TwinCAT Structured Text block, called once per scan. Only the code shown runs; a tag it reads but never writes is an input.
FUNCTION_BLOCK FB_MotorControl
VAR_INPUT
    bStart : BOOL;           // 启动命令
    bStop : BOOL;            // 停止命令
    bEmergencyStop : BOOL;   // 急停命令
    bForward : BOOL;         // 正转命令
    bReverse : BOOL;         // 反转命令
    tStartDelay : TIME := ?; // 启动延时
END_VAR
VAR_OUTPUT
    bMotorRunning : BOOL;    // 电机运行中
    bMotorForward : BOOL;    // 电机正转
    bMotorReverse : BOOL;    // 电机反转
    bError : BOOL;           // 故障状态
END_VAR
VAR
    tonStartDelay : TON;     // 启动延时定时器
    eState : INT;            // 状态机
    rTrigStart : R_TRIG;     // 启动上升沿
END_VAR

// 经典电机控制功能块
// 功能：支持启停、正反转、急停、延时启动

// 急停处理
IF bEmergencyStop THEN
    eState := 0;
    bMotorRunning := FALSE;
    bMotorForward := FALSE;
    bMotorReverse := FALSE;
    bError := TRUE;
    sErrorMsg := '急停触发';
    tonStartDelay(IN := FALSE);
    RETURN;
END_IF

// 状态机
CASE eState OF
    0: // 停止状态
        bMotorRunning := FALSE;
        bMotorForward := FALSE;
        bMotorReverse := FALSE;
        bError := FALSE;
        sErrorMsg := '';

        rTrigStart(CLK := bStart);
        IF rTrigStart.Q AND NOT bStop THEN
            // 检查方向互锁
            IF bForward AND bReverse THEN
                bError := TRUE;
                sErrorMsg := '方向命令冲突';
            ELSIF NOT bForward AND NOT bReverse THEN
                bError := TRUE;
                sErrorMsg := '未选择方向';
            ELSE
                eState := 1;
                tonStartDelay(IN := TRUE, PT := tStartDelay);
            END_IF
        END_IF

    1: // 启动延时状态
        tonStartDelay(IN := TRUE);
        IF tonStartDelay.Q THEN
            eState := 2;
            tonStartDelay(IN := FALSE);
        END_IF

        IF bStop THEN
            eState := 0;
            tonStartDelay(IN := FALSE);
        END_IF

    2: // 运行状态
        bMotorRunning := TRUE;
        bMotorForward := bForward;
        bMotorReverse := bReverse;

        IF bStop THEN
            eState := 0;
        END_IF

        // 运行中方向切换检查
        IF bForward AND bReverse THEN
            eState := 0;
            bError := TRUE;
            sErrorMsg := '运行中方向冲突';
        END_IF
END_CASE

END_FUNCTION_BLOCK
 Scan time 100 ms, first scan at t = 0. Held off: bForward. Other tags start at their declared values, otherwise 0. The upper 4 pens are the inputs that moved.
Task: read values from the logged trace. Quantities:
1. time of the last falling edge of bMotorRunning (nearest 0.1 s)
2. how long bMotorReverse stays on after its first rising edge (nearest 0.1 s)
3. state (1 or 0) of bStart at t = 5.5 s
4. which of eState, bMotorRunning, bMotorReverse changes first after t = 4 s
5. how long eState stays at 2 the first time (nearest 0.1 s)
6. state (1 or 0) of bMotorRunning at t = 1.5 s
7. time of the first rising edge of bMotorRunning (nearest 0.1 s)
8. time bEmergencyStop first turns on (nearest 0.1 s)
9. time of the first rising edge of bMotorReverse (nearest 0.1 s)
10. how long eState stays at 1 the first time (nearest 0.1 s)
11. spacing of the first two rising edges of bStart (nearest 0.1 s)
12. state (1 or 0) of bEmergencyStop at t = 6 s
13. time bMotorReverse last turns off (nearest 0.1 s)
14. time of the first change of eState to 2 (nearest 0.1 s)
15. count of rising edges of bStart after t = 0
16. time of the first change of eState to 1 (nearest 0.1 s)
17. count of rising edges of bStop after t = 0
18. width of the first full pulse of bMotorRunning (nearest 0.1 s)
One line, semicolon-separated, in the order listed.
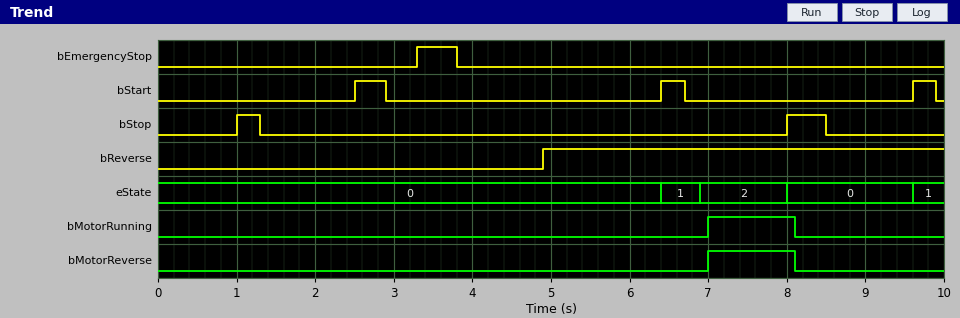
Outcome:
8.1 s; 1.1 s; 0; eState; 1.1 s; 0; 7.0 s; 3.3 s; 7.0 s; 0.5 s; 3.9 s; 0; 8.1 s; 6.9 s; 3; 6.4 s; 2; 1.1 s
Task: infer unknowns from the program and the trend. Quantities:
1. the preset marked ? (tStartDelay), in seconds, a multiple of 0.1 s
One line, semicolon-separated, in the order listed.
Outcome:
0.5 s
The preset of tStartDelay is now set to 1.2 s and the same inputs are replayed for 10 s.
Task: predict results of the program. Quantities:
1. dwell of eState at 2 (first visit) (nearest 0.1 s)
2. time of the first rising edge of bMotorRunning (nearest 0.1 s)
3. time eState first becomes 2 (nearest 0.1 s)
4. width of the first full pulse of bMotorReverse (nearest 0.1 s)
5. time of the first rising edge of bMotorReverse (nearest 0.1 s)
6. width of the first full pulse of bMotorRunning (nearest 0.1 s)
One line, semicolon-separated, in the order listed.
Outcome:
0.4 s; 7.7 s; 7.6 s; 0.4 s; 7.7 s; 0.4 s
